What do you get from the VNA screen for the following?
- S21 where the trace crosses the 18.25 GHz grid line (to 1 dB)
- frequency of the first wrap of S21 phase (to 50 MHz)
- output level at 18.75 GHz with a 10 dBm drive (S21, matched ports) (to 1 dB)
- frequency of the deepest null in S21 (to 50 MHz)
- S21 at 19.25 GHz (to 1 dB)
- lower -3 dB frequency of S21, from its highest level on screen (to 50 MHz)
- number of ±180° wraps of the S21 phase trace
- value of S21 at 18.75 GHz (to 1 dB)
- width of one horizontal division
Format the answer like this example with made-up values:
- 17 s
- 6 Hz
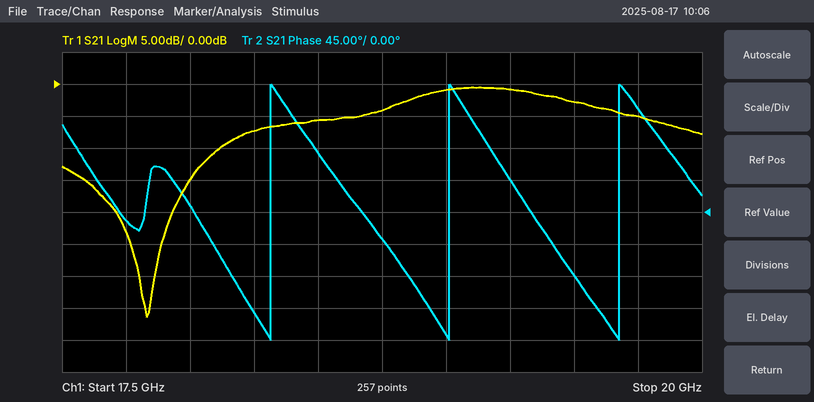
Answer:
- -7 dB
- 18.30 GHz
- 6 dBm
- 17.85 GHz
- -1 dB
- 18.80 GHz
- 3
- -4 dB
- 250 MHz
